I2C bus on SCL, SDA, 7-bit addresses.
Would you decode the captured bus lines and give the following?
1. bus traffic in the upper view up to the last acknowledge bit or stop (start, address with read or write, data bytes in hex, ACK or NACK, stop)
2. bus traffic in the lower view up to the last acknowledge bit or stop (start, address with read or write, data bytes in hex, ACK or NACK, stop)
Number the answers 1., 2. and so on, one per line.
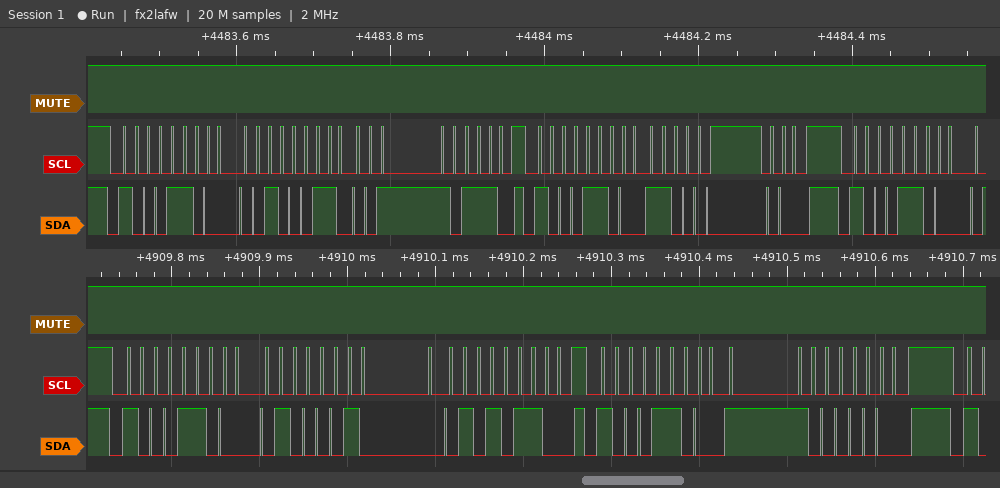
1. start, address 46 write ACK, 23 ACK, 37 ACK, stop, start, address 46 write ACK, C0 ACK, stop, start, address 46 write ACK
2. start, address 46 write ACK, 42 ACK, 56 ACK, stop, start, address 46 write ACK, C0 ACK, stop
